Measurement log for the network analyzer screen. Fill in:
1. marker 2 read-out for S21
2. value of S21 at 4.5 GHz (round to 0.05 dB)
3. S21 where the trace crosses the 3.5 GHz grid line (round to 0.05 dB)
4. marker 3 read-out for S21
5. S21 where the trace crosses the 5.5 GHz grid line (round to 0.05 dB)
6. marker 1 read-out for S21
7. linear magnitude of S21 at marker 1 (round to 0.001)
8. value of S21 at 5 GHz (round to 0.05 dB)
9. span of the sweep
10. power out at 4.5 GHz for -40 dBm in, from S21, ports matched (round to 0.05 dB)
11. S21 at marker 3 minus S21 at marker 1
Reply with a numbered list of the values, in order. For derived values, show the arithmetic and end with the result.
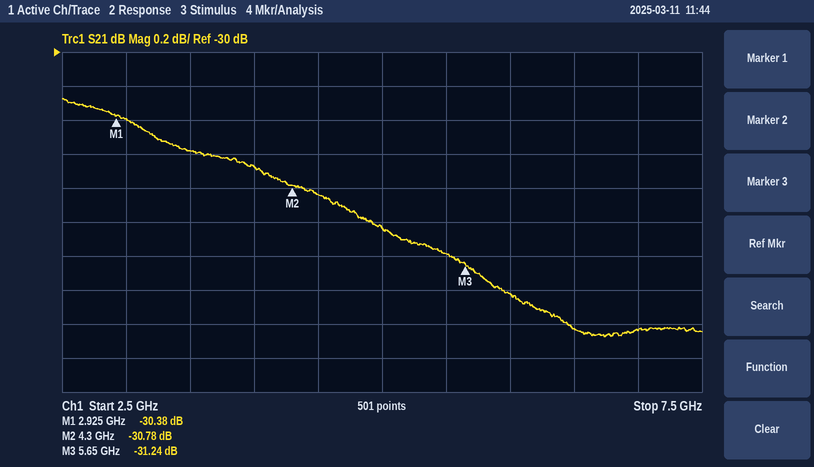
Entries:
1. -30.78 dB
2. -30.85 dB
3. -30.60 dB
4. -31.24 dB
5. -31.20 dB
6. -30.38 dB
7. 10^(-30.38/20) ≈ 0.030
8. -31.05 dB
9. 5 GHz
10. -40 dBm + (-30.85 dB) = -70.85 dBm
11. -31.24 − (-30.38) = -0.86 dB
